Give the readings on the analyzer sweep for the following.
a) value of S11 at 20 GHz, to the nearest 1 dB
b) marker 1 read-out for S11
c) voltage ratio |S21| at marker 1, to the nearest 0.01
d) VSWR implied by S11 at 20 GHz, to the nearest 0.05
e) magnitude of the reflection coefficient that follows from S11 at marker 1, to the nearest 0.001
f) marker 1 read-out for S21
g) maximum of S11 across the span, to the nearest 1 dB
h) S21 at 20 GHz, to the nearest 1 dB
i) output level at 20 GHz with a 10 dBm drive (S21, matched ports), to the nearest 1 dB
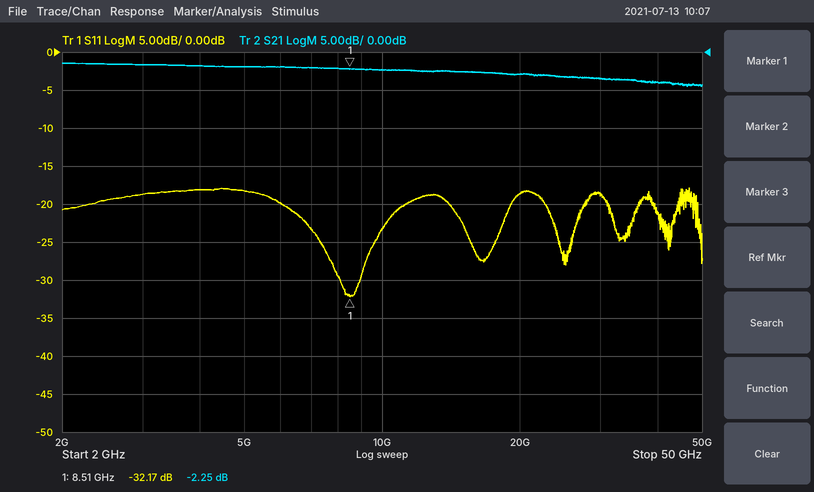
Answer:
-19 dB
-32.17 dB
0.77
1.25
0.025
-2.25 dB
-18 dB
-3 dB
7 dBm
